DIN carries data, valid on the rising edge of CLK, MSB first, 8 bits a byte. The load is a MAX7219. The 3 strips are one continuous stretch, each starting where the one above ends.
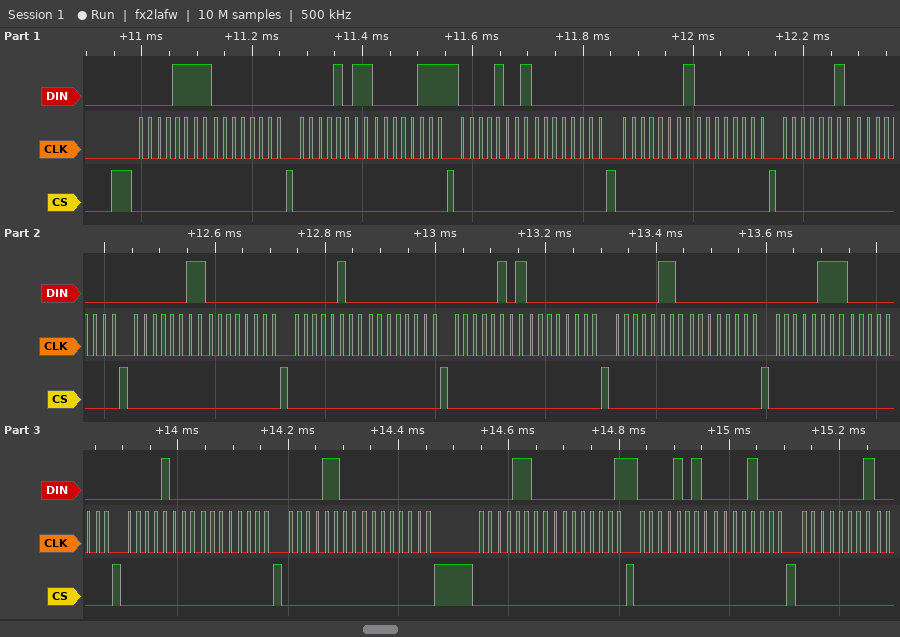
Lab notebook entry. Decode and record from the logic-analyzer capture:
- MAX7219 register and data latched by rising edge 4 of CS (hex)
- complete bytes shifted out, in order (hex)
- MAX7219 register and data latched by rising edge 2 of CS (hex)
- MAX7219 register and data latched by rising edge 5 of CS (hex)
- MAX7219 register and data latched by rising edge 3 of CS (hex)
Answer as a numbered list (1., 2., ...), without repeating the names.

1. register 0x9, data 0x00
2. 0F 00 0B 07 09 00 01 00 02 00 03 00 04 00 05 00 06 00 07 00 08 00 0C 00 0C 01 0A 08 01
3. register 0xF, data 0x00
4. register 0x1, data 0x00
5. register 0xB, data 0x07
